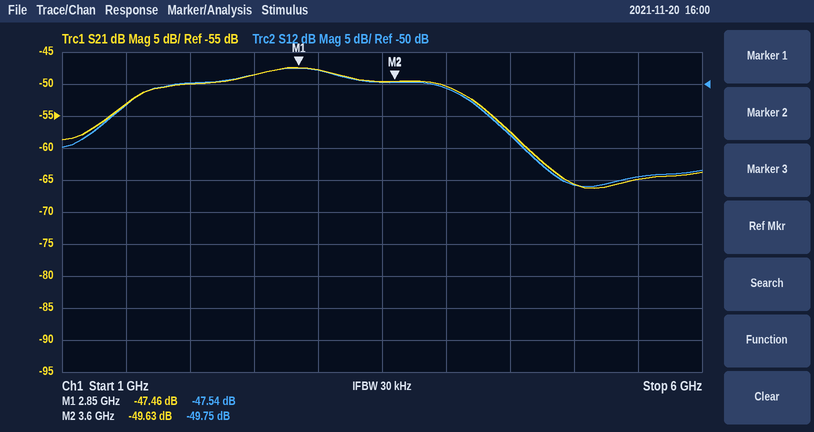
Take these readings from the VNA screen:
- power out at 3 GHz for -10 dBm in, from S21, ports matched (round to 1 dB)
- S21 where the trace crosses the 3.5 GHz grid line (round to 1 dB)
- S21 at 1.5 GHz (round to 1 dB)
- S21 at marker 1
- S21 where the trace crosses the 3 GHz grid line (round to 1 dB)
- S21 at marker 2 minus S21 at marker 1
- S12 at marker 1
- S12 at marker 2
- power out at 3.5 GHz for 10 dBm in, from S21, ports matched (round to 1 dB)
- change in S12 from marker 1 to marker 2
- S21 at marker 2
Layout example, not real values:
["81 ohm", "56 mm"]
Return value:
["-58 dBm", "-50 dB", "-53 dB", "-47.46 dB", "-48 dB", "-2.17 dB", "-47.54 dB", "-49.75 dB", "-40 dBm", "-2.21 dB", "-49.63 dB"]
